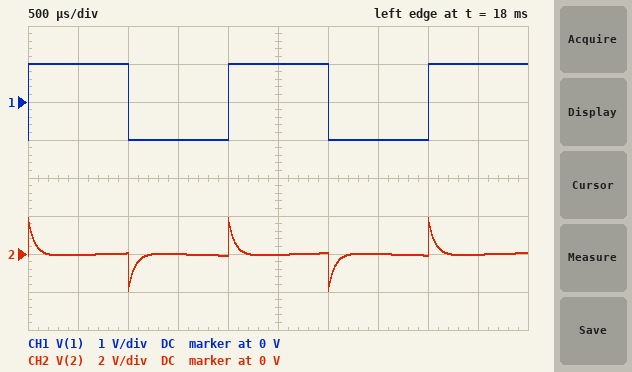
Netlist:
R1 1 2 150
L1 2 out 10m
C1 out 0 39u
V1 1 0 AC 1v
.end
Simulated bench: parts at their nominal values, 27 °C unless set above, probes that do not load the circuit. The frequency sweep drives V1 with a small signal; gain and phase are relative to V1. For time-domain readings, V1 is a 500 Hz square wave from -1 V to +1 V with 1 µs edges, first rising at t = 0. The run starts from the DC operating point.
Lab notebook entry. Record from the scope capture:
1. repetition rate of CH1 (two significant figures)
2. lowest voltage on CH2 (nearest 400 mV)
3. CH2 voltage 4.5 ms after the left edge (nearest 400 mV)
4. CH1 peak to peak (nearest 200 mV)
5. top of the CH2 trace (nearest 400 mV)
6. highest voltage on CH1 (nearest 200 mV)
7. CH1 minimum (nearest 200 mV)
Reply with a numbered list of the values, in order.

1. 500 Hz
2. -2.0 V
3. 0 V
4. 2.0 V
5. 2.0 V
6. 1.0 V
7. -1.0 V
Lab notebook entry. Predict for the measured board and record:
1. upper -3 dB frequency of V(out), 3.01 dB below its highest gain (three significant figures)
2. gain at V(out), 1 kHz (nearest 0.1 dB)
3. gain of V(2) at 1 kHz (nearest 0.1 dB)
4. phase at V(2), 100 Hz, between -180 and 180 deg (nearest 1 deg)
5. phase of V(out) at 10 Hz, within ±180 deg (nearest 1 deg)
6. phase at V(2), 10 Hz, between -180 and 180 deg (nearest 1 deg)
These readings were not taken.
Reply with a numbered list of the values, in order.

1. 27.5 Hz
2. -31.9 dB
3. -8.8 dB
4. -77 deg
5. -20 deg
6. -20 deg
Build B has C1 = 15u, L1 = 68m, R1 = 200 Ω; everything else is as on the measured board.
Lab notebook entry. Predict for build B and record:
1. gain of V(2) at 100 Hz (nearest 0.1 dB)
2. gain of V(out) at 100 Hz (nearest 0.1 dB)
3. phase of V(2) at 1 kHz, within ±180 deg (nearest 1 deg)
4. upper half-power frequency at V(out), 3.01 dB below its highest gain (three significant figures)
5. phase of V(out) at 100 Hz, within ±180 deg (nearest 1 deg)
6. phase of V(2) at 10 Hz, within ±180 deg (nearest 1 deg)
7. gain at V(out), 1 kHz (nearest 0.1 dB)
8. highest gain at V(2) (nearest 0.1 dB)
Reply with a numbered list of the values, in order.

1. -10.4 dB
2. -5.9 dB
3. 26 deg
4. 59.7 Hz
5. -72 deg
6. -11 deg
7. -32.8 dB
8. 0 dB
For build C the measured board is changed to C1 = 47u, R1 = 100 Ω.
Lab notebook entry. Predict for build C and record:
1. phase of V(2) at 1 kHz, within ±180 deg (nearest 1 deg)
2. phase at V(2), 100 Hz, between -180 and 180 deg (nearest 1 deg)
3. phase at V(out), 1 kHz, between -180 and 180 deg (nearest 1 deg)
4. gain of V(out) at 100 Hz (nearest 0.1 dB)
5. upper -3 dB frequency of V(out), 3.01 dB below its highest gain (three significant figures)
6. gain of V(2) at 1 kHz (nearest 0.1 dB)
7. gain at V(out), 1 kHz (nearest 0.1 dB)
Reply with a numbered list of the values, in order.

1. 59 deg
2. -75 deg
3. -121 deg
4. -9.7 dB
5. 34.6 Hz
6. -5.8 dB
7. -30.7 dB
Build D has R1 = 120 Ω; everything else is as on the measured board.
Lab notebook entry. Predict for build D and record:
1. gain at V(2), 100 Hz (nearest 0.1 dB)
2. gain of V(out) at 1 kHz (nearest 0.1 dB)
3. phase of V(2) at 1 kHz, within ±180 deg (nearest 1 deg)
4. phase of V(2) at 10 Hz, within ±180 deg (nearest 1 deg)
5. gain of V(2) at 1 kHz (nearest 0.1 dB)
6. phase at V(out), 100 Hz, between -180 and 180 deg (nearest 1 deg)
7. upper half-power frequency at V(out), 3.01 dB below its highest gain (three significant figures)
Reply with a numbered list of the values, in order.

1. -11.2 dB
2. -30.3 dB
3. 64 deg
4. -16 deg
5. -7.1 dB
6. -74 deg
7. 34.6 Hz
